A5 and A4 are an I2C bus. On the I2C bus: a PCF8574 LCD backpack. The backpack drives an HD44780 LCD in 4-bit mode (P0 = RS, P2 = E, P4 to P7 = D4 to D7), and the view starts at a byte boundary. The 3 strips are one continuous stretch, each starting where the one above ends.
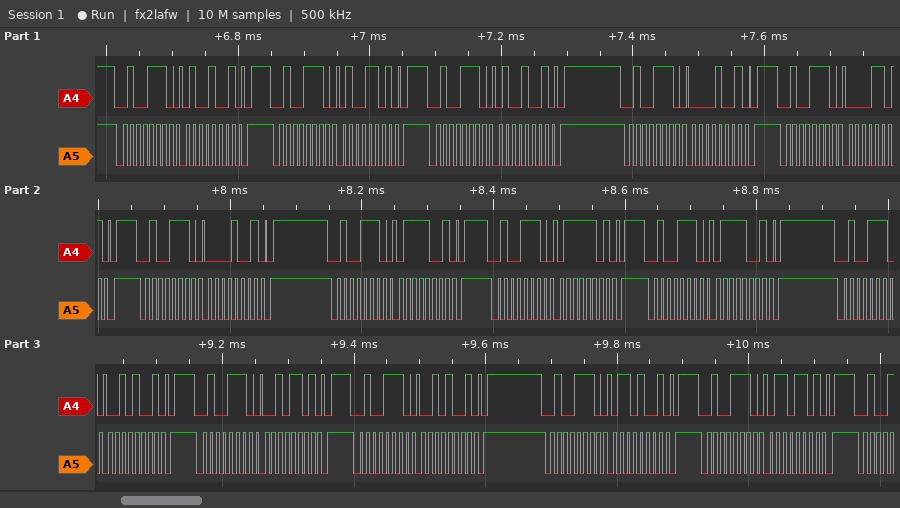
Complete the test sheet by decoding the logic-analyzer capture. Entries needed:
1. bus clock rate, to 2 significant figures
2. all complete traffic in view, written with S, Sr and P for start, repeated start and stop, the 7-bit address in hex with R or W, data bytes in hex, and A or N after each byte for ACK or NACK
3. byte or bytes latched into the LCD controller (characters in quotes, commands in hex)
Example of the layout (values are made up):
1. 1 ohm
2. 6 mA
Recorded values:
1. 100 kHz
2. S 27W A 49 A P S 27W A 4D A P S 27W A 49 A P S 27W A 09 A P S 27W A 0D A P S 27W A 09 A P S 27W A 79 A P S 27W A 7D A P S 27W A 79 A P S 27W A 29 A P S 27W A 2D A P S 27W A 29 A P S 27W A 69 A P S 27W A 6D A P
3. '@' 'r'
